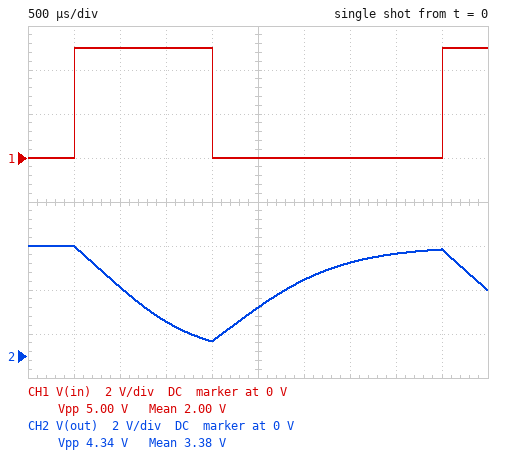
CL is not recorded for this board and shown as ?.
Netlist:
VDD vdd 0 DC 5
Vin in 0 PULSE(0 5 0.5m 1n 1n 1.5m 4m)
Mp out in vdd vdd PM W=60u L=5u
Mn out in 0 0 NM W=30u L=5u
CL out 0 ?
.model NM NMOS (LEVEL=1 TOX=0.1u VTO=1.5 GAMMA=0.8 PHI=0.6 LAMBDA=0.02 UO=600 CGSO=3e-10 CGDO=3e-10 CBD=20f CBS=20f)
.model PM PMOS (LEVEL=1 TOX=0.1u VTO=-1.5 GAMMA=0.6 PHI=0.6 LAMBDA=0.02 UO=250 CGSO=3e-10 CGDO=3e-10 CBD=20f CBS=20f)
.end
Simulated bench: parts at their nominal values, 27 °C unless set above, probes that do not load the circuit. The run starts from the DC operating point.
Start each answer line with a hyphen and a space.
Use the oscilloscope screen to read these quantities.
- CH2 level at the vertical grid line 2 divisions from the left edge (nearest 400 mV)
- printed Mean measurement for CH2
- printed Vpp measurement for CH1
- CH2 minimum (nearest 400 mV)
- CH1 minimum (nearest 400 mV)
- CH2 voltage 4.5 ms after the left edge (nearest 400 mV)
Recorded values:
- 3.2 V
- 3.38 V
- 5.00 V
- 800 mV
- 0 V
- 4.8 V
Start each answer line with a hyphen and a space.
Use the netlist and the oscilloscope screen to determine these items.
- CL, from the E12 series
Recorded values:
- 220 nF
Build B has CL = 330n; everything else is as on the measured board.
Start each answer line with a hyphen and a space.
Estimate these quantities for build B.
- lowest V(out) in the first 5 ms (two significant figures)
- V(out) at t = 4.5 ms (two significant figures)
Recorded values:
- 1.6 V
- 4.6 V
